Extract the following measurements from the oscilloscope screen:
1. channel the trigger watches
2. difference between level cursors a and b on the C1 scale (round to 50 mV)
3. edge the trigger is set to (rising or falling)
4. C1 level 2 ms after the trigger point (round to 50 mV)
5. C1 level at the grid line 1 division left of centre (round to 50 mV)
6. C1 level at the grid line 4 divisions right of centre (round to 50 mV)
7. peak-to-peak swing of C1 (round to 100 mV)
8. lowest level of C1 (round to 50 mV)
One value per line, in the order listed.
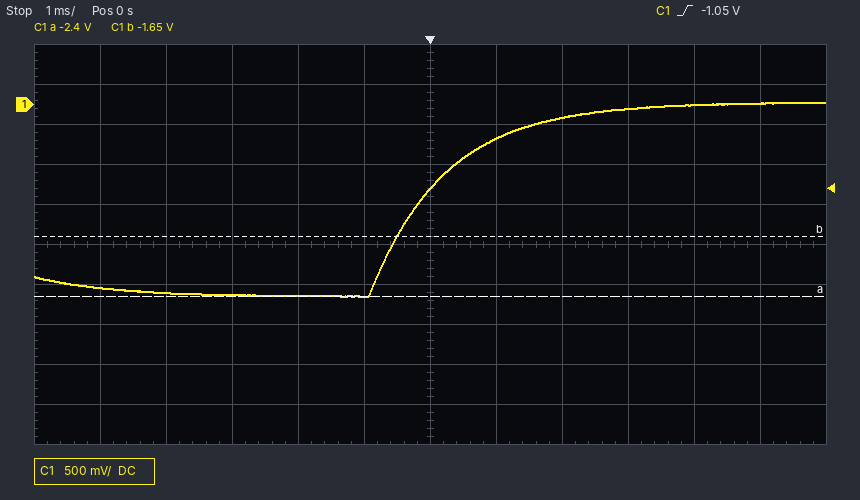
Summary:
C1
750 mV
rising
-150 mV
-2.40 V
0 mV
2.40 V
-2.40 V
